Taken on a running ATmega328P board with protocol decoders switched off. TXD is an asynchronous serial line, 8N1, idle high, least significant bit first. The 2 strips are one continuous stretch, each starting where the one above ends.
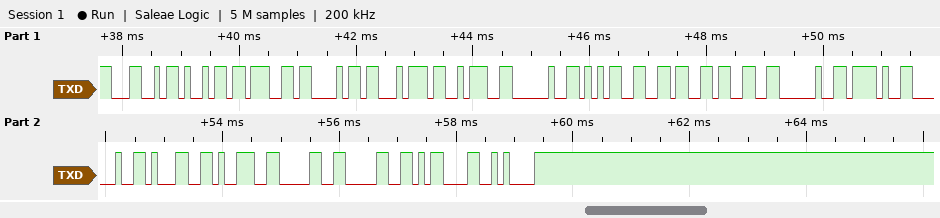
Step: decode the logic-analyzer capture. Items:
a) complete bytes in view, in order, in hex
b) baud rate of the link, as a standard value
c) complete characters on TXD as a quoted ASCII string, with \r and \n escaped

0x4C 0x69 0x67 0x68 0x74 0x3A 0x20 0x35 0x36 0x33 0x20 0x2F 0x20 0x31 0x39 0x30 0x30 0x0D 0x0A
9600 baud
"Light: 563 / 1900\r\n"
